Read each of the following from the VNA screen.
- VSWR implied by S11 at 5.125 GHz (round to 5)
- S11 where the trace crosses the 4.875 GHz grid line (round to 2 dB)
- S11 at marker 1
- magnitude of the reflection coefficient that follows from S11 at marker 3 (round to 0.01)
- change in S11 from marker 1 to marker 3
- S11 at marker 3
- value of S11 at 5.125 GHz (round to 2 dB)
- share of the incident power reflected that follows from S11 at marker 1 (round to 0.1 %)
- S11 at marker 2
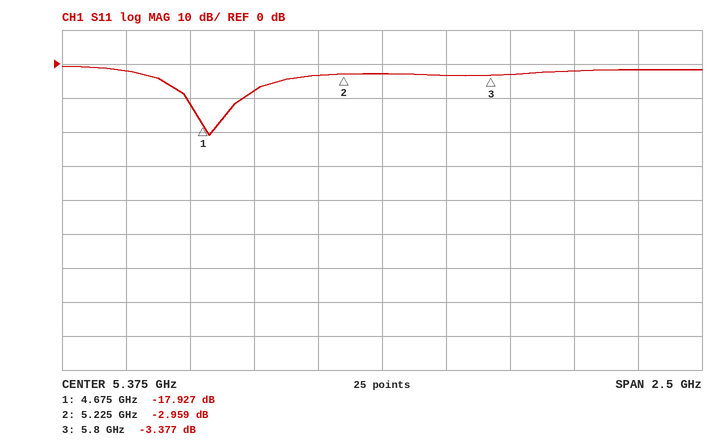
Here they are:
5
-8 dB
-17.927 dB
0.68
14.550 dB
-3.377 dB
-4 dB
1.6 %
-2.959 dB
